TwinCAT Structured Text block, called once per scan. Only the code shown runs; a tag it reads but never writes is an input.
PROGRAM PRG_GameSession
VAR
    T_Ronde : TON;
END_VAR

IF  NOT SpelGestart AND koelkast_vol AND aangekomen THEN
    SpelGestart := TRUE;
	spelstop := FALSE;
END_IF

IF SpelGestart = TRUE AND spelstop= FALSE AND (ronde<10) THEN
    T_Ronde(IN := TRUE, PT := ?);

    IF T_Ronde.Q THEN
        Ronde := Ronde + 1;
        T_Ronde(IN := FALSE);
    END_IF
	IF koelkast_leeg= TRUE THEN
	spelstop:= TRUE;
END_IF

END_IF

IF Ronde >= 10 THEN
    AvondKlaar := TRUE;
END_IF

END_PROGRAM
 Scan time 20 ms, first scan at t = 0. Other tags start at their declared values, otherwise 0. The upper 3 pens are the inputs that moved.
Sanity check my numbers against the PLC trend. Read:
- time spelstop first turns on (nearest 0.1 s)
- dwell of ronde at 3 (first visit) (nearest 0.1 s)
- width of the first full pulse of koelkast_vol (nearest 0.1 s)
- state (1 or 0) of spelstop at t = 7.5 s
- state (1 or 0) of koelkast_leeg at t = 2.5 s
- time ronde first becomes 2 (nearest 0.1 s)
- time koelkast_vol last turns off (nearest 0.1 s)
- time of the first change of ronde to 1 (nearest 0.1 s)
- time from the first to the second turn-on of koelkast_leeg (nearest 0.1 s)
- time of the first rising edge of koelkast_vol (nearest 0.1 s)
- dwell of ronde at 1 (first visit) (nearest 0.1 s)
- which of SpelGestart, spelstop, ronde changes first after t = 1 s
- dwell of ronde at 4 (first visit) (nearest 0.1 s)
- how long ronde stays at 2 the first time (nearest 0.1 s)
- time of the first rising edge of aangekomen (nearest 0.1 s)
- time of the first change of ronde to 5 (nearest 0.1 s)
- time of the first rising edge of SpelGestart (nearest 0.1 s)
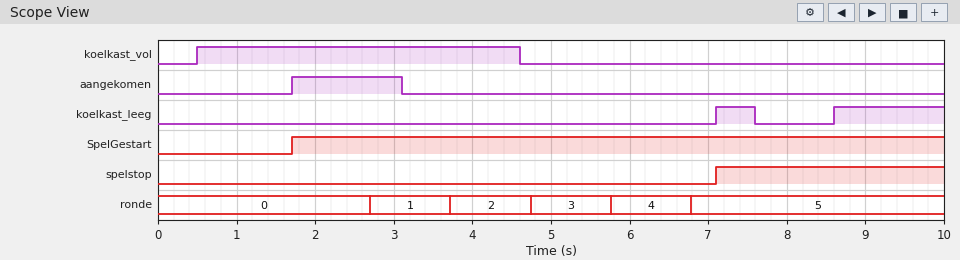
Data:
7.1 s
1.0 s
4.1 s
1
0
3.7 s
4.6 s
2.7 s
1.5 s
0.5 s
1.0 s
SpelGestart
1.0 s
1.0 s
1.7 s
6.8 s
1.7 s
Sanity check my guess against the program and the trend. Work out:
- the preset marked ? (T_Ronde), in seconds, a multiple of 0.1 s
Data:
1.0 s
